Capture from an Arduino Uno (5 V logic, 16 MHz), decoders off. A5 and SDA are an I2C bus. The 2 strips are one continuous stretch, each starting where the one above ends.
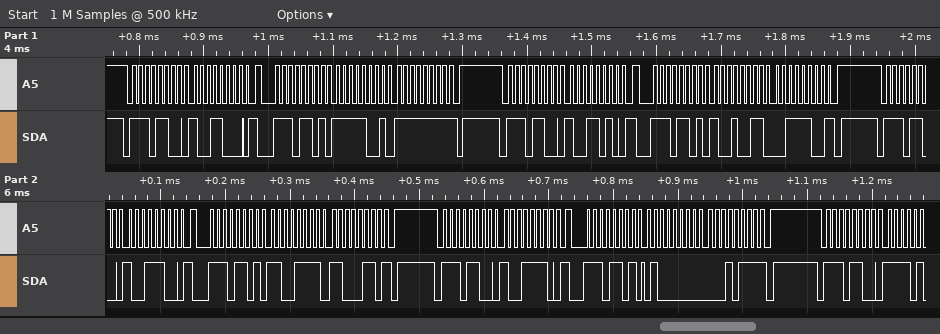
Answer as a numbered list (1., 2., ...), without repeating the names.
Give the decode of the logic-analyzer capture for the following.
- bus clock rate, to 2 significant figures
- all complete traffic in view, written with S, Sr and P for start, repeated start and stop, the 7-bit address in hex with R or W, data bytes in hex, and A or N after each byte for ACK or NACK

1. 100 kHz
2. S 76W A 98 A Sr 76R A F9 A FF N P S 76W A 9A A Sr 76R A 93 A 3C N P S 76W A 9C A Sr 76R A CF A C6 N P S 76W A 9E A Sr 76R A 40 A 17 N P S 76W A
